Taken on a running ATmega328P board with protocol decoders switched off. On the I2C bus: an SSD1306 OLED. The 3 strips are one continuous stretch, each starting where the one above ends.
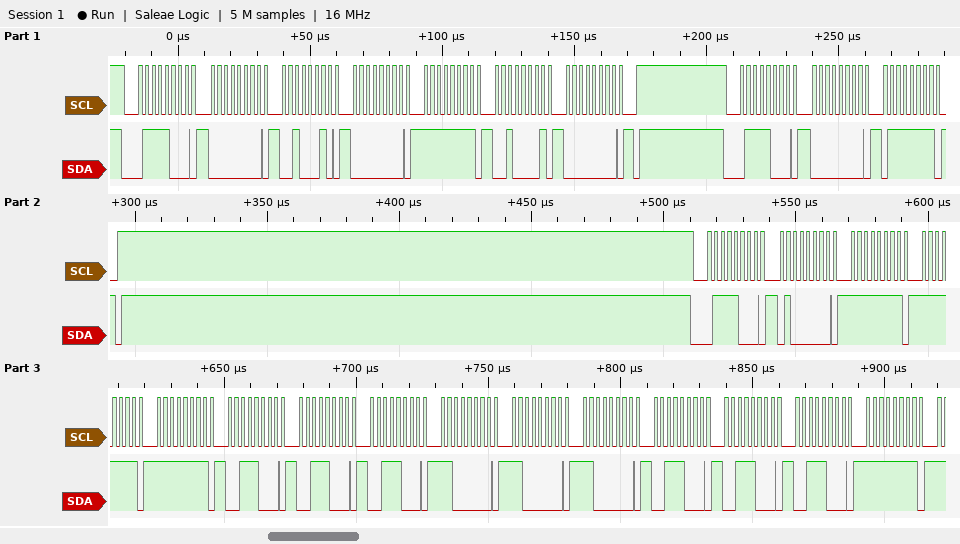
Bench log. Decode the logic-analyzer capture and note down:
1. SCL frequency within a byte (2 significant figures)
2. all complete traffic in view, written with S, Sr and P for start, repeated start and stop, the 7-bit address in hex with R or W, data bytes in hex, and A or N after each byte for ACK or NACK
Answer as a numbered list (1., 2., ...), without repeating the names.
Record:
1. 400 kHz
2. S 3CW A 00 A 22 A 00 A FF A 21 A 00 A P S 3CW A 00 A 7F A P S 3CW A 40 A FF A FF A FF A 38 A 38 A 38 A C0 A C0 A C0 A 38 A 38 A 38 A FF A
